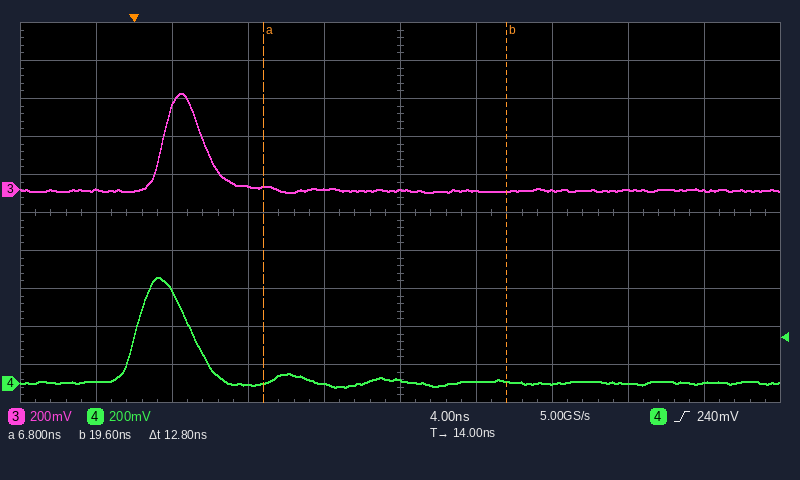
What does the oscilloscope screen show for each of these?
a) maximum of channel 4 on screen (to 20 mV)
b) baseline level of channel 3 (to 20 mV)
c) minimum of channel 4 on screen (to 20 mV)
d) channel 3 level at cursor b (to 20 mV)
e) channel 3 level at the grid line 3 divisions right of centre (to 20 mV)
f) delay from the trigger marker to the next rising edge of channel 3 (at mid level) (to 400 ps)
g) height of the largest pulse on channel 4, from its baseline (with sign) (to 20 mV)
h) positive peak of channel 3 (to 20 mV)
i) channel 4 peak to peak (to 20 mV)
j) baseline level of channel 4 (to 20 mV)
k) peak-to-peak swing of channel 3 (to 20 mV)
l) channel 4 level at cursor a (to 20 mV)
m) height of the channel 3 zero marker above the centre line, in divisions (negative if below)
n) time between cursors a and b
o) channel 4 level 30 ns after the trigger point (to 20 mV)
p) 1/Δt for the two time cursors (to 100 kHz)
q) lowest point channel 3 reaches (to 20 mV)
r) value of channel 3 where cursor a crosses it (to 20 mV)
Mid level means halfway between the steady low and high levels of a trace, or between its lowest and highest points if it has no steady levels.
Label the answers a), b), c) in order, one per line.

a) 560 mV
b) 0 mV
c) -20 mV
d) 0 mV
e) 0 mV
f) 1.6 ns
g) +560 mV
h) 500 mV
i) 580 mV
j) 0 mV
k) 520 mV
l) 0 mV
m) +0.6 div
n) 12.8 ns
o) 0 mV
p) 78.1 MHz
q) -20 mV
r) 20 mV
